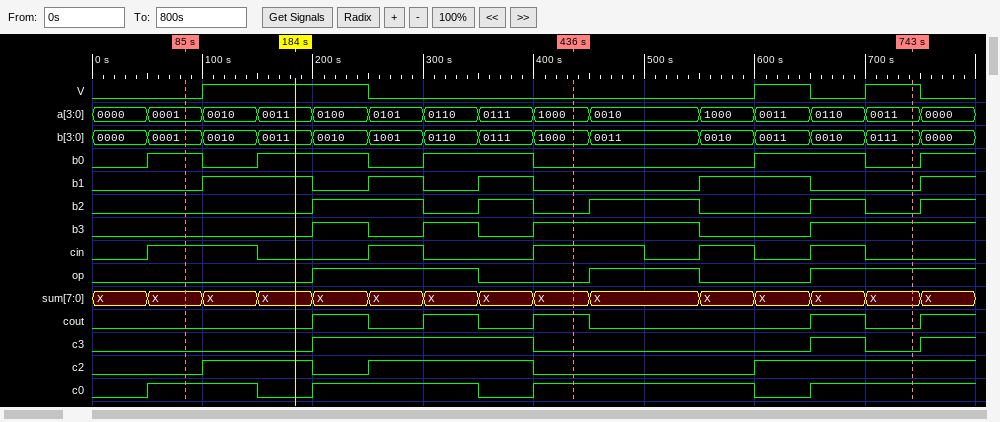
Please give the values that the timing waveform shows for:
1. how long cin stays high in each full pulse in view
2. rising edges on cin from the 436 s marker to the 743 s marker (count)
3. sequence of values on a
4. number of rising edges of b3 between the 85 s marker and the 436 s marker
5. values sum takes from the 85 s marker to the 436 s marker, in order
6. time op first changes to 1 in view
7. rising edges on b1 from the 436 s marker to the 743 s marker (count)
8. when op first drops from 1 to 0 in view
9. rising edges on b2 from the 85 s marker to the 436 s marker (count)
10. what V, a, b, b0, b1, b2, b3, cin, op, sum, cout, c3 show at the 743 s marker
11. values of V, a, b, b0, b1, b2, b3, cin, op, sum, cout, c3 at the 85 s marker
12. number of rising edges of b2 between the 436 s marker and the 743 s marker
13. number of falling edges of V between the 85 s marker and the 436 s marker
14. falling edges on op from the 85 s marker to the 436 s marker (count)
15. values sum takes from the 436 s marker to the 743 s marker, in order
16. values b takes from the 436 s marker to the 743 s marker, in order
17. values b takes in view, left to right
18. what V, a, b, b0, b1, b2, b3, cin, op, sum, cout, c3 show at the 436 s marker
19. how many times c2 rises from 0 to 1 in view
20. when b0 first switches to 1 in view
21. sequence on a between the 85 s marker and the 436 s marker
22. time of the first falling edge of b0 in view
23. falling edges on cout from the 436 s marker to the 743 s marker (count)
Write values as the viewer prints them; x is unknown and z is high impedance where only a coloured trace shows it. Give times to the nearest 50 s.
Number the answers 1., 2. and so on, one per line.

1. 100 s, 50 s, 100 s, 50 s, 50 s
2. 2
3. 0000, 0001, 0010, 0011, 0100, 0101, 0110, 0111, 1000, 0010, 1000, 0011, 0110, 0011, 0000
4. 3
5. X, X, X, X, X, X, X, X
6. 200 s
7. 1
8. 350 s
9. 2
10. V=1, a=0011, b=0111, b0=0, b1=0, b2=0, b3=1, cin=0, op=1, sum=X, cout=0, c3=0
11. V=0, a=0001, b=0001, b0=1, b1=0, b2=0, b3=0, cin=1, op=0, sum=X, cout=0, c3=0
12. 2
13. 1
14. 1
15. X, X, X, X, X, X
16. 1000, 0011, 0010, 0011, 0010, 0111
17. 0000, 0001, 0010, 0011, 0010, 1001, 0110, 0111, 1000, 0011, 0010, 0011, 0010, 0111, 0000
18. V=0, a=1000, b=1000, b0=0, b1=0, b2=0, b3=1, cin=1, op=0, sum=X, cout=1, c3=0
19. 3
20. 50 s
21. 0001, 0010, 0011, 0100, 0101, 0110, 0111, 1000
22. 100 s
23. 2
